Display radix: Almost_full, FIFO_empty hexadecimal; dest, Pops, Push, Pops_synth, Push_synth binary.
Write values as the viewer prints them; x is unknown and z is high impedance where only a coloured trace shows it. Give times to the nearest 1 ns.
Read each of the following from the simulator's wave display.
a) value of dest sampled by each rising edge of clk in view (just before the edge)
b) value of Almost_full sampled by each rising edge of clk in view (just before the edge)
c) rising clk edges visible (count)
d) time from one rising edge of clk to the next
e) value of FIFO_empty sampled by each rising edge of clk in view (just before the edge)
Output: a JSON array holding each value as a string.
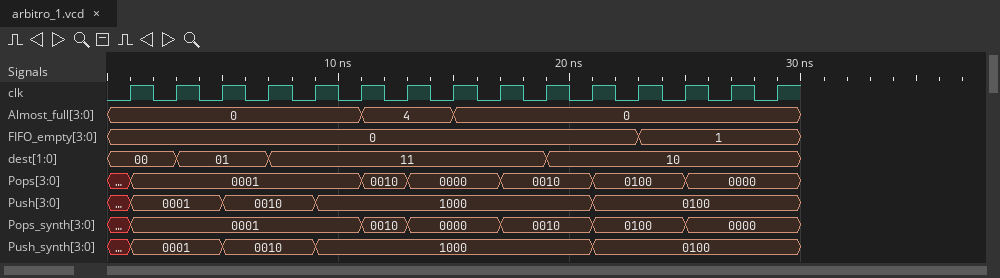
["00, 00, 01, 01, 11, 11, 11, 11, 11, 11, 10, 10, 10, 10, 10", "0, 0, 0, 0, 0, 0, 4, 4, 0, 0, 0, 0, 0, 0, 0", "15", "2 ns", "0, 0, 0, 0, 0, 0, 0, 0, 0, 0, 0, 0, 1, 1, 1"]
